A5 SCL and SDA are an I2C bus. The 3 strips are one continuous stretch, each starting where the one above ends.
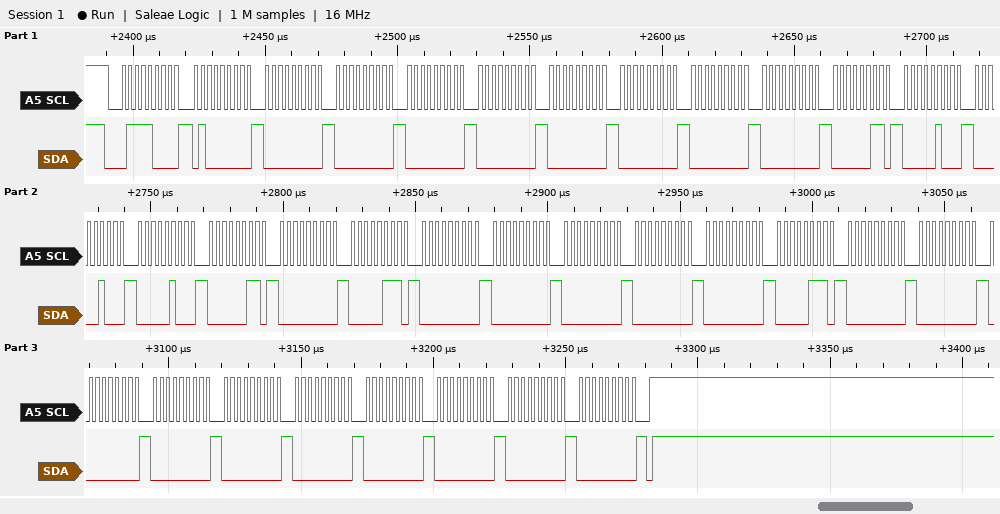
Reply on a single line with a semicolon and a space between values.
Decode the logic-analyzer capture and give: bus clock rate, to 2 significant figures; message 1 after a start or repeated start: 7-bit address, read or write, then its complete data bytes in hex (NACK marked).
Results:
400 kHz; 0x3C write: 40 00 00 00 00 00 00 00 00 03 04 04 04 03 00 07 00 00 00 00 00 07 00 00 00 00 00 00 00 00 00 00
